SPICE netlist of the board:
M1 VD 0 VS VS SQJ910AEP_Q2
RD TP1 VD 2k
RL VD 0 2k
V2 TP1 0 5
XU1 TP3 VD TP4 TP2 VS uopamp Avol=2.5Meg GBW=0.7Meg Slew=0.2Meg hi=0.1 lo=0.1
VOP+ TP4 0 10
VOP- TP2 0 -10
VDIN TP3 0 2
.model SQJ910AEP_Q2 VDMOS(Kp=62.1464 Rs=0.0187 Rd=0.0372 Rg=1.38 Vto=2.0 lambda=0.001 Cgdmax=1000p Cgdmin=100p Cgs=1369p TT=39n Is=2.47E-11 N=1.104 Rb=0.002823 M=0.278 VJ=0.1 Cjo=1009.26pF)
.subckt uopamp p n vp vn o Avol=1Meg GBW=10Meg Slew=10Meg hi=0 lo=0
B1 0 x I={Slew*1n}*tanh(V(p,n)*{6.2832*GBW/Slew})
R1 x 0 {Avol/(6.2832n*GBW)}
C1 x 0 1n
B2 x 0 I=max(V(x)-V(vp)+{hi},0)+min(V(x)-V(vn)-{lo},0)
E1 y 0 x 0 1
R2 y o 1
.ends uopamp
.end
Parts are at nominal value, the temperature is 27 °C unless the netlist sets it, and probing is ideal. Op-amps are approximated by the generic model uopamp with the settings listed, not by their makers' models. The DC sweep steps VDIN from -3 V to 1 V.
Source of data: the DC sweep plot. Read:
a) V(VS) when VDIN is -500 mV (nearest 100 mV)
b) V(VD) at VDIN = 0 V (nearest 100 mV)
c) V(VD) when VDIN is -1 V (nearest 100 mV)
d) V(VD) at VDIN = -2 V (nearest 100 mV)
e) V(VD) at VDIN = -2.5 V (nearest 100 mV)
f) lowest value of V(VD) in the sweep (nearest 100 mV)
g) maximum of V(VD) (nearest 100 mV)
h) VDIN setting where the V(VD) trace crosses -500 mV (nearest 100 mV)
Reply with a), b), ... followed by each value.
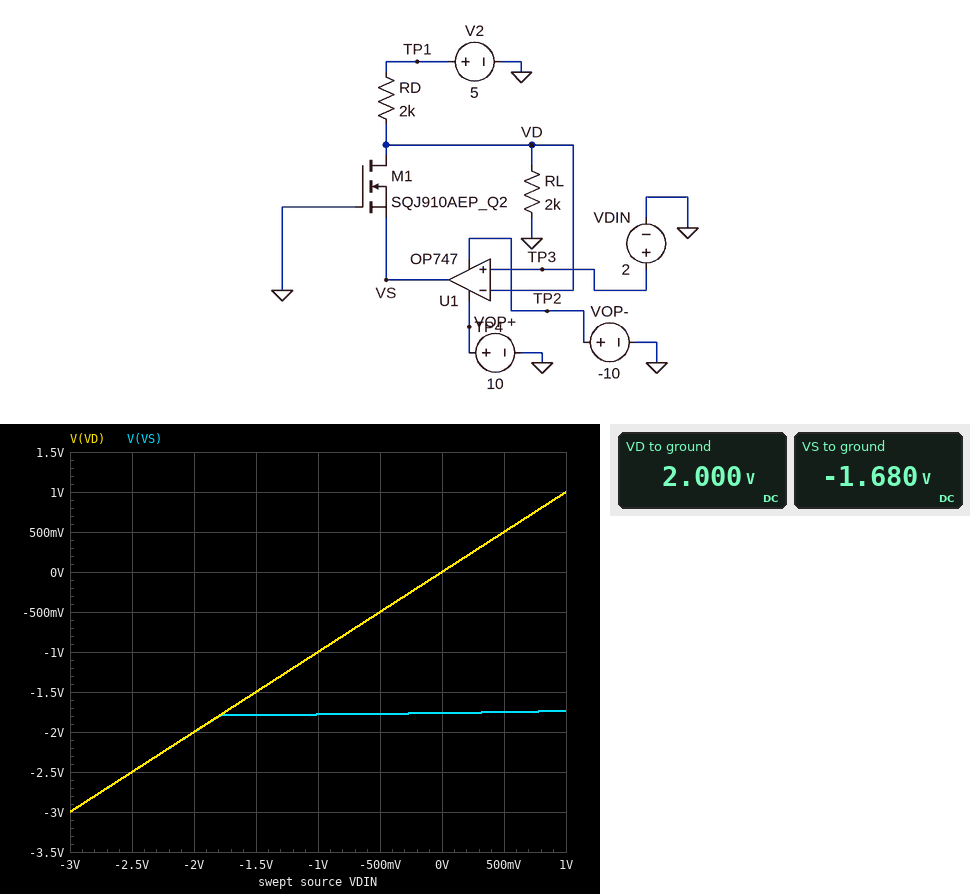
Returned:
a) -1.8 V
b) 0 V
c) -1.0 V
d) -2.0 V
e) -2.5 V
f) -3.0 V
g) 1.0 V
h) -500 mV
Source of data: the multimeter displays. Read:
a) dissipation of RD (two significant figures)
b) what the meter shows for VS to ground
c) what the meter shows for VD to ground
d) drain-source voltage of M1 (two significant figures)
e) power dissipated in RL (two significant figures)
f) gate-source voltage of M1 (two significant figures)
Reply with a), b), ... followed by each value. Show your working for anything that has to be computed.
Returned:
a) (5 V - 2 V)^2 / 2 kΩ = 4.5 mW
b) -1.680 V
c) 2.000 V
d) 2 V - (-1.68 V) = 3.7 V
e) (2 V)^2 / 2 kΩ = 2.0 mW
f) 0 V - (-1.68 V) = 1.7 V
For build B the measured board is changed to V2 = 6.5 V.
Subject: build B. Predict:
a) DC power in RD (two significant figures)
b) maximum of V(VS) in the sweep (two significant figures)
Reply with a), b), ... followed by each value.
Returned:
a) 10 mW
b) -1.8 V
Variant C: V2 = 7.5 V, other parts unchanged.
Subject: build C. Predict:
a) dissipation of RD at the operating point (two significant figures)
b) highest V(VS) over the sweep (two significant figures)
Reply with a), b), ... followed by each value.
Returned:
a) 15 mW
b) -1.8 V
